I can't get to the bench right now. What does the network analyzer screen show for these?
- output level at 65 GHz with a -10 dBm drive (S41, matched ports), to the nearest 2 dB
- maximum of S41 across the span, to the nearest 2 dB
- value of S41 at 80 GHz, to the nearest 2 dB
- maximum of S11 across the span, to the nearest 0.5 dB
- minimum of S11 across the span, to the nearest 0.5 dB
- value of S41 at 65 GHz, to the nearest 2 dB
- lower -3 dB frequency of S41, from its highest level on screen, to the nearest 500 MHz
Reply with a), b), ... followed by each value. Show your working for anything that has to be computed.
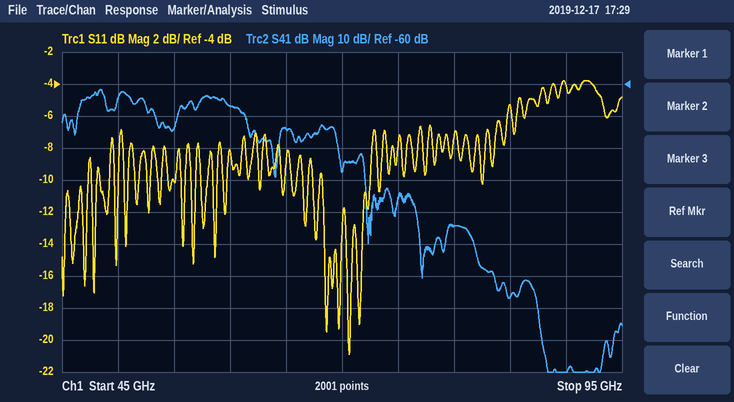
a) -10 dBm + (-74 dB) = -84 dBm
b) -62 dB
c) -104 dB
d) -4.0 dB
e) -21.0 dB
f) -74 dB
g) 47.0 GHz
